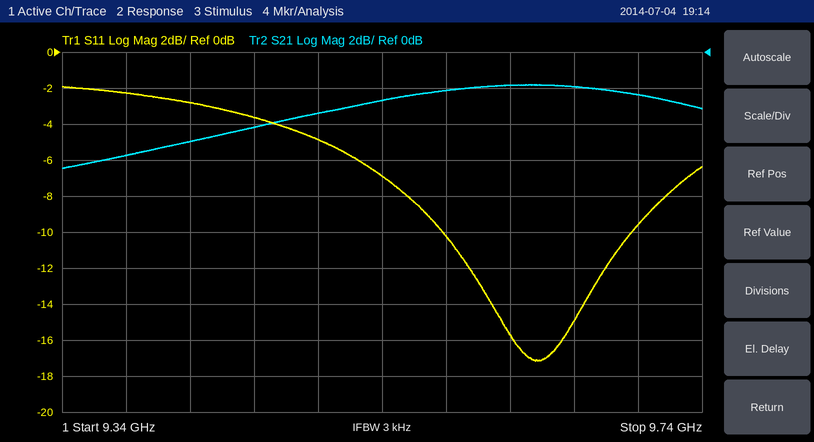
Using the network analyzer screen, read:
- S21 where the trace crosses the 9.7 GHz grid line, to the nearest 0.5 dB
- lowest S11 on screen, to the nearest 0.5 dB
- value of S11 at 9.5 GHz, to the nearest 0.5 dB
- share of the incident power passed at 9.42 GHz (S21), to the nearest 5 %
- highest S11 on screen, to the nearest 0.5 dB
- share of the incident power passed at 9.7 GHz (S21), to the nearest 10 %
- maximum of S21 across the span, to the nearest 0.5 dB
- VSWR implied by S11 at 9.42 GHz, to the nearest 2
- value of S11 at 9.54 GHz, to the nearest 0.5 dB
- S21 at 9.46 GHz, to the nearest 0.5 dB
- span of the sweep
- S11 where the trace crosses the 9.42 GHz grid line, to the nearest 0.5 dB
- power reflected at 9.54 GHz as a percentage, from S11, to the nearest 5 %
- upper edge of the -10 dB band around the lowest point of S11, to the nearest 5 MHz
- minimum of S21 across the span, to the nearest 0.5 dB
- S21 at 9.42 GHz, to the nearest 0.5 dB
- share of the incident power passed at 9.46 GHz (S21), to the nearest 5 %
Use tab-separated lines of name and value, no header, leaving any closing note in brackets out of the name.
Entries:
S21 where the trace crosses the 9.7 GHz grid line, to the nearest 0.5 dB	-2.5 dB
lowest S11 on screen, to the nearest 0.5 dB	-17.0 dB
value of S11 at 9.5 GHz, to the nearest 0.5 dB	-5.0 dB
share of the incident power passed at 9.42 GHz (S21), to the nearest 5 %	30 %
highest S11 on screen, to the nearest 0.5 dB	-2.0 dB
share of the incident power passed at 9.7 GHz (S21), to the nearest 10 %	60 %
maximum of S21 across the span, to the nearest 0.5 dB	-2.0 dB
VSWR implied by S11 at 9.42 GHz, to the nearest 2	6
value of S11 at 9.54 GHz, to the nearest 0.5 dB	-7.0 dB
S21 at 9.46 GHz, to the nearest 0.5 dB	-4.0 dB
span of the sweep	400 MHz
S11 where the trace crosses the 9.42 GHz grid line, to the nearest 0.5 dB	-3.0 dB
power reflected at 9.54 GHz as a percentage, from S11, to the nearest 5 %	20 %
upper edge of the -10 dB band around the lowest point of S11, to the nearest 5 MHz	9.695 GHz
minimum of S21 across the span, to the nearest 0.5 dB	-6.5 dB
S21 at 9.42 GHz, to the nearest 0.5 dB	-5.0 dB
share of the incident power passed at 9.46 GHz (S21), to the nearest 5 %	40 %
